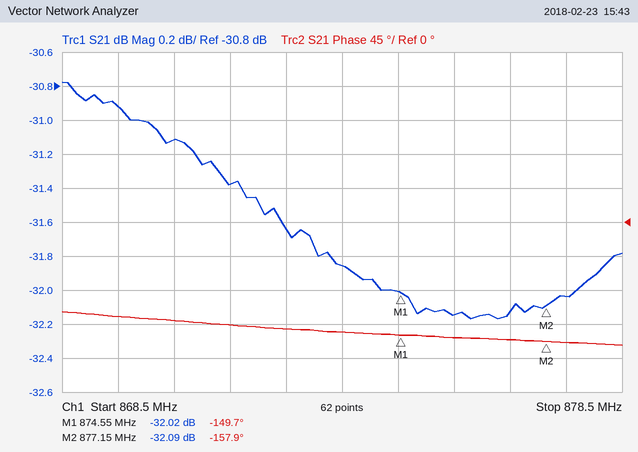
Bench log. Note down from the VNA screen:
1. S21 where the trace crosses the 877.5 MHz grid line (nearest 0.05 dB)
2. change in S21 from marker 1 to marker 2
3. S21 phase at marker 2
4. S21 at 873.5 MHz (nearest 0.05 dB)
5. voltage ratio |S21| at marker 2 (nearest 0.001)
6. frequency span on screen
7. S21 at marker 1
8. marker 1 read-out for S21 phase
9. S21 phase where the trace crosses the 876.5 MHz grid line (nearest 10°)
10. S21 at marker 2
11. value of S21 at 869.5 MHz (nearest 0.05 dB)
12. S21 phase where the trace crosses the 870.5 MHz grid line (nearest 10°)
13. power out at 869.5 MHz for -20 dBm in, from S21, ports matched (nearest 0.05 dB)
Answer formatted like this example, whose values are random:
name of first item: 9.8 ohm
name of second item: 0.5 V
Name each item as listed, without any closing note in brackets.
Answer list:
S21 where the trace crosses the 877.5 MHz grid line: -32.05 dB
change in S21 from marker 1 to marker 2: -0.07 dB
S21 phase at marker 2: -157.9°
S21 at 873.5 MHz: -31.85 dB
voltage ratio |S21| at marker 2: 0.025
frequency span on screen: 10 MHz
S21 at marker 1: -32.02 dB
marker 1 read-out for S21 phase: -149.7°
S21 phase where the trace crosses the 876.5 MHz grid line: -160°
S21 at marker 2: -32.09 dB
value of S21 at 869.5 MHz: -30.90 dB
S21 phase where the trace crosses the 870.5 MHz grid line: -130°
power out at 869.5 MHz for -20 dBm in, from S21, ports matched: -50.90 dBm
